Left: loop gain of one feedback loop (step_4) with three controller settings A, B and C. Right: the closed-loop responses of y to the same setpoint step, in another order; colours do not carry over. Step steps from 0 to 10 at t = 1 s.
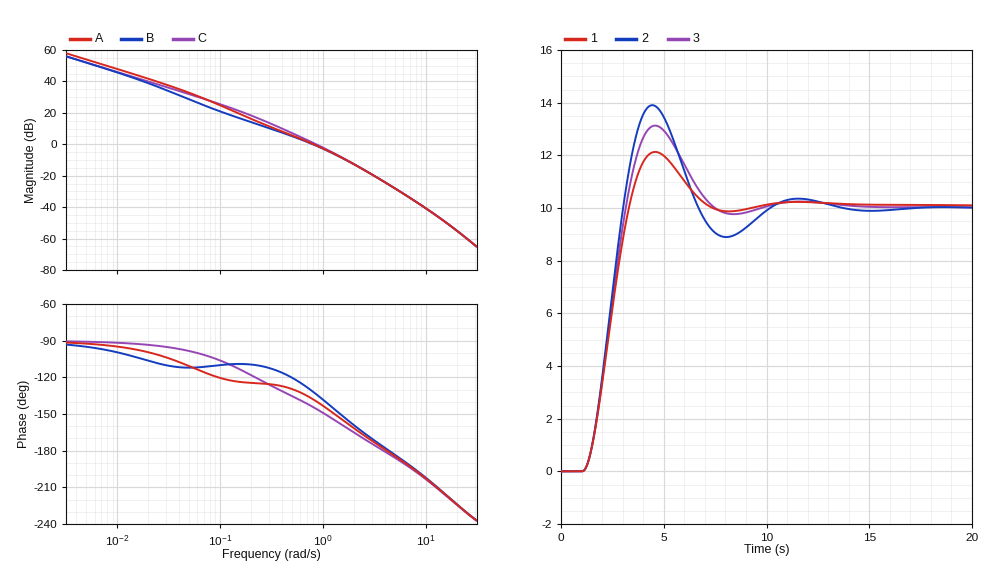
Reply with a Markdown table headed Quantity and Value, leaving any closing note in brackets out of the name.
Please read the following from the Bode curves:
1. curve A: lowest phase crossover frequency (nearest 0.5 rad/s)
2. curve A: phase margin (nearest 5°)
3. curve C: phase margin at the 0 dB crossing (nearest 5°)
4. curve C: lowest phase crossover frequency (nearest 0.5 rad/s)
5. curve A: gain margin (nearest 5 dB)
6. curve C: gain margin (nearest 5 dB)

| Quantity | Value |
|---|---|
| curve A: lowest phase crossover frequency | 4.0 rad/s |
| curve A: phase margin | 40° |
| curve C: phase margin at the 0 dB crossing | 35° |
| curve C: lowest phase crossover frequency | 4.0 rad/s |
| curve A: gain margin | 25 dB |
| curve C: gain margin | 25 dB |
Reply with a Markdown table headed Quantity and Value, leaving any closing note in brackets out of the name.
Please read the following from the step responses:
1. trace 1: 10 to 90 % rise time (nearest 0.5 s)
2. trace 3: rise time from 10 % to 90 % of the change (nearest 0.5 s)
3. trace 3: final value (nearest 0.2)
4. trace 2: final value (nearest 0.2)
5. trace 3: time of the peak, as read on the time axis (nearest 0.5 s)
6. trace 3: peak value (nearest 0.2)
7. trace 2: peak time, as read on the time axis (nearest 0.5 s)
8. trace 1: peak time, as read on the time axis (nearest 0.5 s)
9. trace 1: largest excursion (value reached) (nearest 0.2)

| Quantity | Value |
|---|---|
| trace 1: 10 to 90 % rise time | 1.5 s |
| trace 3: rise time from 10 % to 90 % of the change | 1.5 s |
| trace 3: final value | 10.0 |
| trace 2: final value | 10.0 |
| trace 3: time of the peak, as read on the time axis | 4.5 s |
| trace 3: peak value | 13.2 |
| trace 2: peak time, as read on the time axis | 4.5 s |
| trace 1: peak time, as read on the time axis | 4.5 s |
| trace 1: largest excursion (value reached) | 12.2 |
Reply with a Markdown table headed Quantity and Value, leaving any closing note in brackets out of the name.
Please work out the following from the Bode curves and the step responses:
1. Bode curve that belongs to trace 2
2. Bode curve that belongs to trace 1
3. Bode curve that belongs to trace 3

| Quantity | Value |
|---|---|
| Bode curve that belongs to trace 2 | C |
| Bode curve that belongs to trace 1 | B |
| Bode curve that belongs to trace 3 | A |
